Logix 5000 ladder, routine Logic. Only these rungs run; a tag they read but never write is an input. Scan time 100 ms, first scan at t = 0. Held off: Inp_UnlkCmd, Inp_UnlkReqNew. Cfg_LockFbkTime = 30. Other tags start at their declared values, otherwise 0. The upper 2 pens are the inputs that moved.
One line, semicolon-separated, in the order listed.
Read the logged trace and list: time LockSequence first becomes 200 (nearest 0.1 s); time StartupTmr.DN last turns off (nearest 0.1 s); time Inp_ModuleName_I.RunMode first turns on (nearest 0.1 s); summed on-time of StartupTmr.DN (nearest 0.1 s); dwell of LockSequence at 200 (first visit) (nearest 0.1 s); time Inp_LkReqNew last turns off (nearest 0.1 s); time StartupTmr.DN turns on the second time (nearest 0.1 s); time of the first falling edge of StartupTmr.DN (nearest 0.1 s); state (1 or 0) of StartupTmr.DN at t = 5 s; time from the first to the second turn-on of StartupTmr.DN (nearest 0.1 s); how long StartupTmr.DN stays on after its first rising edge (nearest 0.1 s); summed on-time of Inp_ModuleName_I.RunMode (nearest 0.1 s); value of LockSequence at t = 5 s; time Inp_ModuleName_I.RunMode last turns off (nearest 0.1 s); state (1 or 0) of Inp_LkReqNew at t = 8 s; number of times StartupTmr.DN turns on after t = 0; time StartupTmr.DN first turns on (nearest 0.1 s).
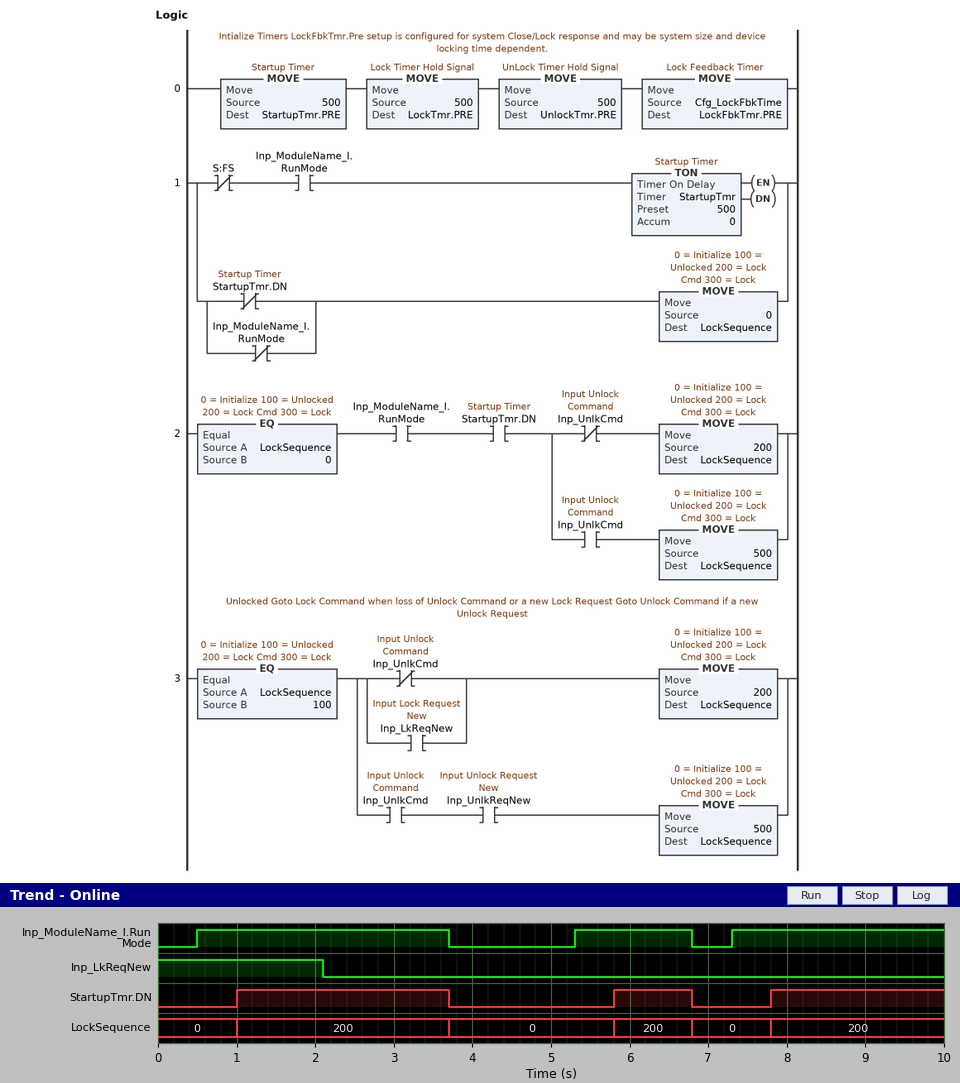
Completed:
1.0 s; 6.8 s; 0.5 s; 5.9 s; 2.7 s; 2.1 s; 5.8 s; 3.7 s; 0; 4.8 s; 2.7 s; 7.4 s; 0; 6.8 s; 0; 3; 1.0 s
